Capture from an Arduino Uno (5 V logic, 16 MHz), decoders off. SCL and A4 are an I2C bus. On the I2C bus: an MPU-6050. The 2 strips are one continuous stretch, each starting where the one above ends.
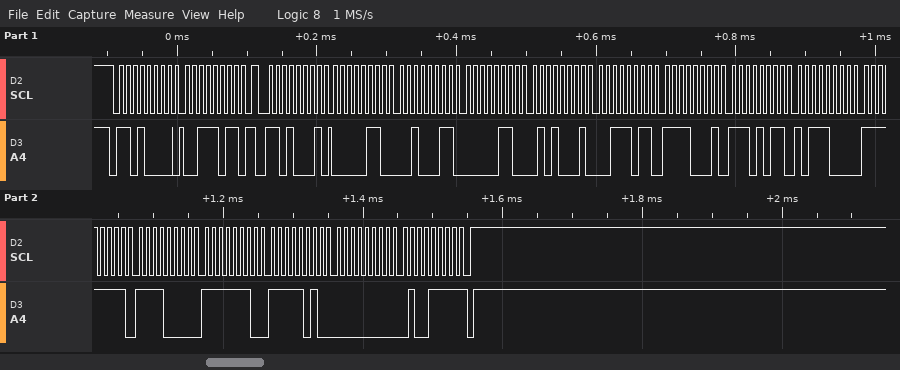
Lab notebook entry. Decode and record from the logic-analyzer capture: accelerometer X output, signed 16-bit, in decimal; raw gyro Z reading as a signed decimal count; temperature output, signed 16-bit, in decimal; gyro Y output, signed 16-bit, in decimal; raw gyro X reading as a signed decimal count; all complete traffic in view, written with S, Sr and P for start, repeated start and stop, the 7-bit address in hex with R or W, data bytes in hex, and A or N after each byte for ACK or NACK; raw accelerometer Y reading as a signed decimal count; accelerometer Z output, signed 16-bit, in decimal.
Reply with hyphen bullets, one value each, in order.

- 1571
- 79
- -5192
- -262
- -16
- S 68W A 3B A Sr 68R A 06 A 23 A 06 A 51 A 3B A F1 A EB A B8 A FF A F0 A FE A FA A 00 A 4F N P
- 1617
- 15345
